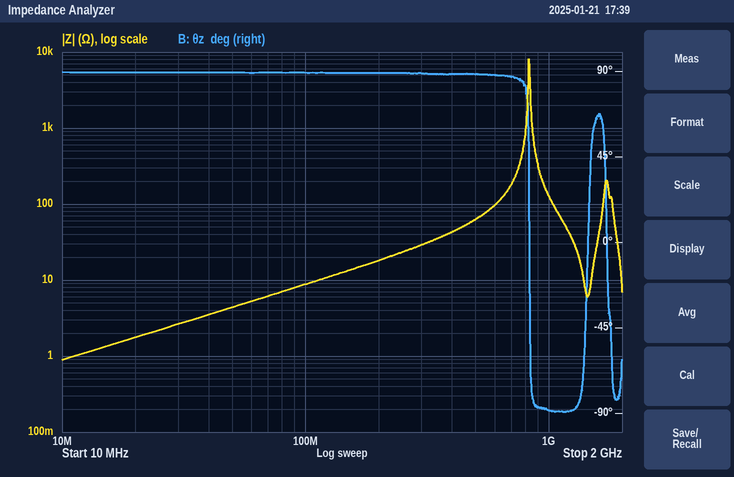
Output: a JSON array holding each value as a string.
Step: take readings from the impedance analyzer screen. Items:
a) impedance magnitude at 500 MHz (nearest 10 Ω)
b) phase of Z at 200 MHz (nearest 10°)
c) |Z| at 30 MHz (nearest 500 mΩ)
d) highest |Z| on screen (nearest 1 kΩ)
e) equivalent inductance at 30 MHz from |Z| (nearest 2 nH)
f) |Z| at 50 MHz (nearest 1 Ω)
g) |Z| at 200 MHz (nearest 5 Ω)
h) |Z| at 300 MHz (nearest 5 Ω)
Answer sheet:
["60 Ω", "90°", "2.5 Ω", "8 kΩ", "14 nH", "4 Ω", "20 Ω", "30 Ω"]
